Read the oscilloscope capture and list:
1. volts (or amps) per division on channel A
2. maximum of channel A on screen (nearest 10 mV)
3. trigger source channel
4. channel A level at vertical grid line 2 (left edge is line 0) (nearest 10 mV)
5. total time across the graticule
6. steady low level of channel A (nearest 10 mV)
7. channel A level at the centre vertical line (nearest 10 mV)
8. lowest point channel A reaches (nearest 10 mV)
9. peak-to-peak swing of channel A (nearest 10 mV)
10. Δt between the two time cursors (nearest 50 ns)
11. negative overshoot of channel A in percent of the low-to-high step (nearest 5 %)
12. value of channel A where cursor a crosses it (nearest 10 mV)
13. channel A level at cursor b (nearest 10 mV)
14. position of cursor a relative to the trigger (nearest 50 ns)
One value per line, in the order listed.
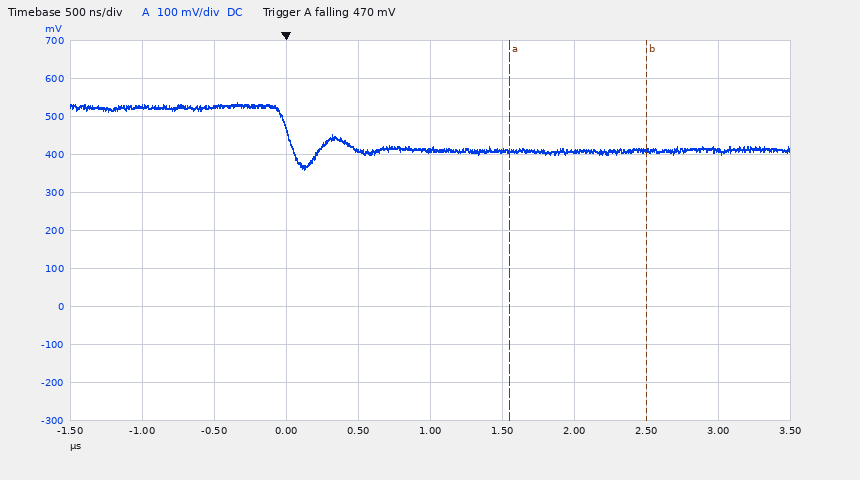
100 mV
540 mV
channel A
520 mV
5 µs
410 mV
410 mV
360 mV
180 mV
950 ns
45 %
410 mV
410 mV
+1.55 µs
